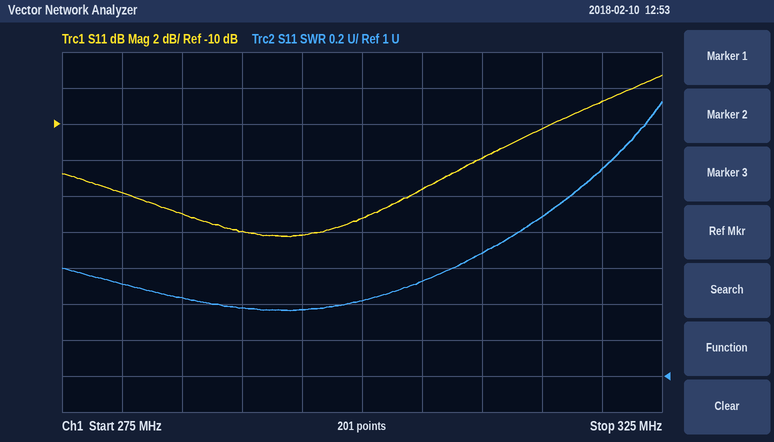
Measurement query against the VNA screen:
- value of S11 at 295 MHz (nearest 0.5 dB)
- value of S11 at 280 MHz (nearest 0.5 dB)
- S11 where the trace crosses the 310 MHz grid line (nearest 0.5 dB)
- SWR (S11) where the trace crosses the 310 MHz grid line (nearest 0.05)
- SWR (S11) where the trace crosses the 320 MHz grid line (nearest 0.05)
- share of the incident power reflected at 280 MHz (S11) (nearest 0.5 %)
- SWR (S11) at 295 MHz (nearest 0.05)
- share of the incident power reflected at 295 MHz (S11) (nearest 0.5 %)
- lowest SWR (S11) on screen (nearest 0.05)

-16.0 dB
-14.0 dB
-12.0 dB
1.70
2.15
4.0 %
1.35
2.5 %
1.35
